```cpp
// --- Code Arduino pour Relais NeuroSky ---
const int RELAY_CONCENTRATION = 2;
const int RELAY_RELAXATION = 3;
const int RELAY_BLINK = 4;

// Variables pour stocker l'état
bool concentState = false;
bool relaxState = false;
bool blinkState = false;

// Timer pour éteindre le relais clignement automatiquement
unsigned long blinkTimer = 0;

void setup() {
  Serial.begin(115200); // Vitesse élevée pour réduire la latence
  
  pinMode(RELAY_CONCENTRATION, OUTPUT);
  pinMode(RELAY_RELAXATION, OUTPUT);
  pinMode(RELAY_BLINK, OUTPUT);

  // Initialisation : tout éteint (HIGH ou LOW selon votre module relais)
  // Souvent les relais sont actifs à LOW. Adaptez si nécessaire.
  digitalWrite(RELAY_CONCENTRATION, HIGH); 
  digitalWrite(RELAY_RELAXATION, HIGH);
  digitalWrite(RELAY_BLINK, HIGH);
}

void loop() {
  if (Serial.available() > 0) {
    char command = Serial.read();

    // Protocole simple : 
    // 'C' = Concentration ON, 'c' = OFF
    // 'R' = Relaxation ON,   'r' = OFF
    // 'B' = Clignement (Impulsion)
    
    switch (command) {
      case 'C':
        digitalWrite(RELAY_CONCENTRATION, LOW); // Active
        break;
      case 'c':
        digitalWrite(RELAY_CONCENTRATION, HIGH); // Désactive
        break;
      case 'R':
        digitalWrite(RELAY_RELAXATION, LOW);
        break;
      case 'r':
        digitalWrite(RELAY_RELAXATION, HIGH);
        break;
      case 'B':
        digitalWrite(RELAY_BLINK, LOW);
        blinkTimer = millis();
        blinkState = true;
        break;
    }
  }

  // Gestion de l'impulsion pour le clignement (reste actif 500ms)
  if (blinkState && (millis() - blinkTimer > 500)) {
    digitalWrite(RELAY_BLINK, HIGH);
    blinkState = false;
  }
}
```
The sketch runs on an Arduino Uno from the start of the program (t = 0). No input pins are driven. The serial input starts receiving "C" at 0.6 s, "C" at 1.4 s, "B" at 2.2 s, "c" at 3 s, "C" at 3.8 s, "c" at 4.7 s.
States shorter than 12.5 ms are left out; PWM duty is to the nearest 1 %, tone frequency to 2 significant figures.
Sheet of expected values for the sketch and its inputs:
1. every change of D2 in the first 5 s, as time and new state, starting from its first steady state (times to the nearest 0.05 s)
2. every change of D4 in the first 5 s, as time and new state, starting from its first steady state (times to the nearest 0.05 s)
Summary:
0 s high; 0.6 s low; 3 s high; 3.8 s low; 4.7 s high
0 s high; 2.2 s low; 2.7 s high
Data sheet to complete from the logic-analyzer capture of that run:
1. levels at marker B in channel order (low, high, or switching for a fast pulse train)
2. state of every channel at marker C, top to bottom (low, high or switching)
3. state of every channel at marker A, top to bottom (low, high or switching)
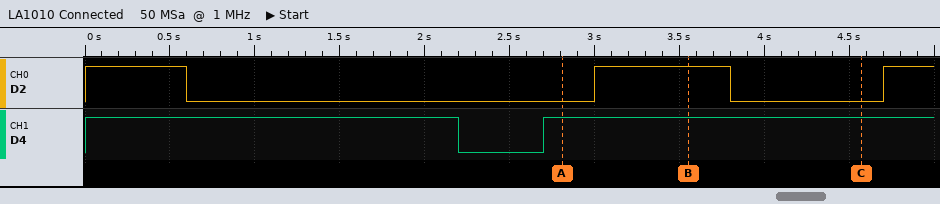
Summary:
D2 high, D4 high
D2 low, D4 high
D2 low, D4 high
